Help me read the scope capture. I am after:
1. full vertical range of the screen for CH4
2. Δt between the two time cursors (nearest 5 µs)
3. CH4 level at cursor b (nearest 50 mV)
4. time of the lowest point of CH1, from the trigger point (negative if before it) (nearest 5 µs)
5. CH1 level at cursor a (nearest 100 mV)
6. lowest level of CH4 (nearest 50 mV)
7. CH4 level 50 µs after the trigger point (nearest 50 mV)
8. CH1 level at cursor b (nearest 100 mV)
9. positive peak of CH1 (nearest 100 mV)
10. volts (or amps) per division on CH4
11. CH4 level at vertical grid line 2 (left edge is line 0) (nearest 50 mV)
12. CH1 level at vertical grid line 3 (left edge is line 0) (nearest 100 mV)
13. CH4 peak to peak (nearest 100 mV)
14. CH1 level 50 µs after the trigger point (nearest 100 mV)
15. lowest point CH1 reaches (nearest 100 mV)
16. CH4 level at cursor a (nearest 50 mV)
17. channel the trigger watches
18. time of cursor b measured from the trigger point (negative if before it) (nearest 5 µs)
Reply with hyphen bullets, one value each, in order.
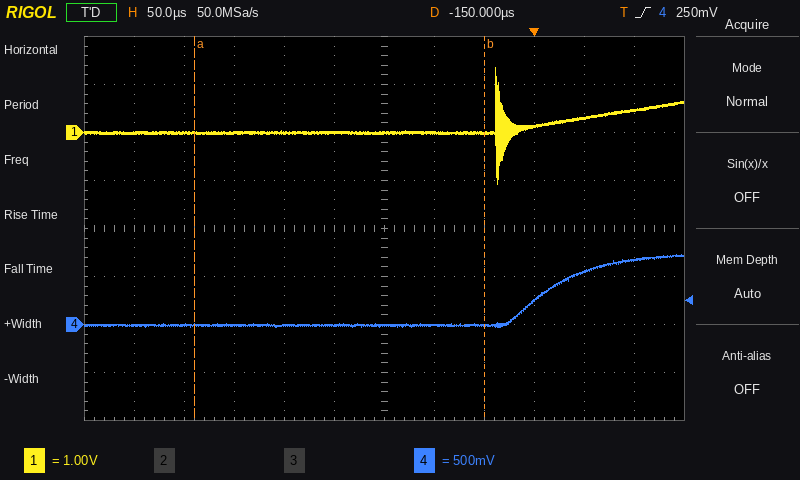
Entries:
- 4 V
- 290 µs
- 0 mV
- -35 µs
- 0.0 V
- -50 mV
- 550 mV
- 0.0 V
- 1.4 V
- 500 mV
- 0 mV
- 0.0 V
- 800 mV
- 300 mV
- -1.1 V
- 0 mV
- CH4
- -50 µs
